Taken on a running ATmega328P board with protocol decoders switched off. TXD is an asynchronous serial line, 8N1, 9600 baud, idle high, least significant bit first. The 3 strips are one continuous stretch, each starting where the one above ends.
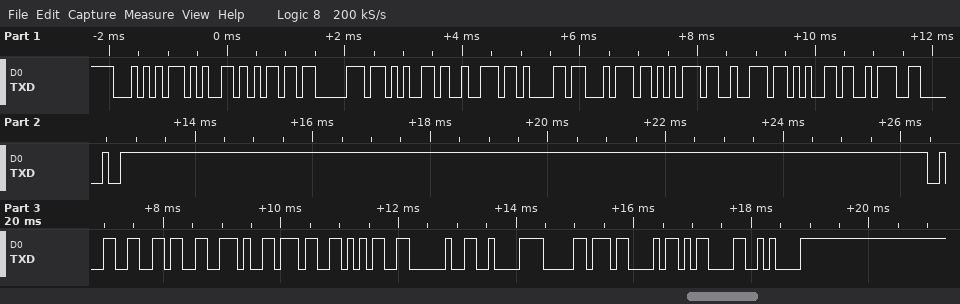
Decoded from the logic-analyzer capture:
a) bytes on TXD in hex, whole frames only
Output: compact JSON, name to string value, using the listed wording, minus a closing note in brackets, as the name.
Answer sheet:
{"bytes on TXD in hex, whole frames only": "0x54 0x65 0x6D 0x70 0x65 0x72 0x61 0x74 0x75 0x72 0x65 0x3A 0x20 0x32 0x36 0x2E 0x37 0x35 0x20 0xC2 0xB0 0x43 0x0D 0x0A"}
